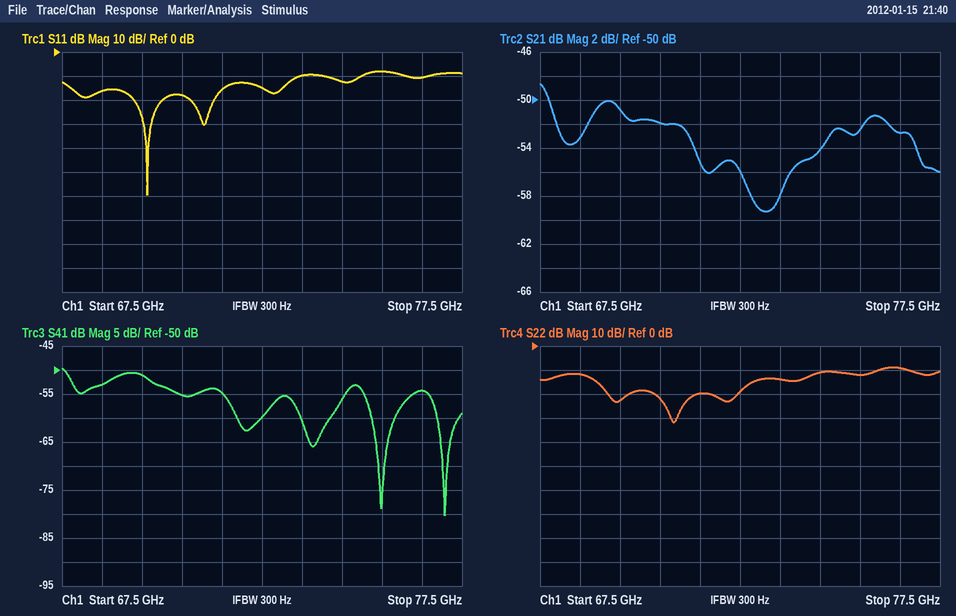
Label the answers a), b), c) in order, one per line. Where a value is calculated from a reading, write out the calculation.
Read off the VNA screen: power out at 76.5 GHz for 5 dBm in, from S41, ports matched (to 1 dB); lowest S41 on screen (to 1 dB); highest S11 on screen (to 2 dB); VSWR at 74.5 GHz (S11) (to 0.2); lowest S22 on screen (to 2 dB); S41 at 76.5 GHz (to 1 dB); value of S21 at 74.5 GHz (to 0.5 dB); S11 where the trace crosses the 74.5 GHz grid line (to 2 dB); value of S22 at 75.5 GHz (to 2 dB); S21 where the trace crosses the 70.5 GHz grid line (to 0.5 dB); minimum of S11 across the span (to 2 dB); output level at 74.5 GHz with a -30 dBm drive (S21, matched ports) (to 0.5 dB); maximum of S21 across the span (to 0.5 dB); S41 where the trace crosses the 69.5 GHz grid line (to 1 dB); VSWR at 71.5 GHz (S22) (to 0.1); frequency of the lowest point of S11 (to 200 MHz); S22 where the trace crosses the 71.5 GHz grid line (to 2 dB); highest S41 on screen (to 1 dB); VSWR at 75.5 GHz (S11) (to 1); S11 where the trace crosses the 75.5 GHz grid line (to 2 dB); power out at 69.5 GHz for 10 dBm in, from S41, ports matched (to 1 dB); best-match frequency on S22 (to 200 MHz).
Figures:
a) 5 dBm + (-54 dB) = -49 dBm
b) -80 dB
c) -8 dB
d) |Γ| = 10^(-12/20) = 0.2512; VSWR = (1 + 0.2512)/(1 − 0.2512) ≈ 1.67, so 1.6 to the nearest 0.2
e) -32 dB
f) -54 dB
g) -54.0 dB
h) -12 dB
i) -12 dB
j) -52.0 dB
k) -60 dB
l) -30 dBm + (-54.0 dB) = -84.0 dBm
m) -48.5 dB
n) -51 dB
o) |Γ| = 10^(-20/20) = 0.1000; VSWR = (1 + 0.1000)/(1 − 0.1000) ≈ 1.2
p) 69.6 GHz
q) -20 dB
r) -50 dB
s) |Γ| = 10^(-8/20) = 0.3981; VSWR = (1 + 0.3981)/(1 − 0.3981) ≈ 2
t) -8 dB
u) 10 dBm + (-51 dB) = -41 dBm
v) 70.8 GHz
